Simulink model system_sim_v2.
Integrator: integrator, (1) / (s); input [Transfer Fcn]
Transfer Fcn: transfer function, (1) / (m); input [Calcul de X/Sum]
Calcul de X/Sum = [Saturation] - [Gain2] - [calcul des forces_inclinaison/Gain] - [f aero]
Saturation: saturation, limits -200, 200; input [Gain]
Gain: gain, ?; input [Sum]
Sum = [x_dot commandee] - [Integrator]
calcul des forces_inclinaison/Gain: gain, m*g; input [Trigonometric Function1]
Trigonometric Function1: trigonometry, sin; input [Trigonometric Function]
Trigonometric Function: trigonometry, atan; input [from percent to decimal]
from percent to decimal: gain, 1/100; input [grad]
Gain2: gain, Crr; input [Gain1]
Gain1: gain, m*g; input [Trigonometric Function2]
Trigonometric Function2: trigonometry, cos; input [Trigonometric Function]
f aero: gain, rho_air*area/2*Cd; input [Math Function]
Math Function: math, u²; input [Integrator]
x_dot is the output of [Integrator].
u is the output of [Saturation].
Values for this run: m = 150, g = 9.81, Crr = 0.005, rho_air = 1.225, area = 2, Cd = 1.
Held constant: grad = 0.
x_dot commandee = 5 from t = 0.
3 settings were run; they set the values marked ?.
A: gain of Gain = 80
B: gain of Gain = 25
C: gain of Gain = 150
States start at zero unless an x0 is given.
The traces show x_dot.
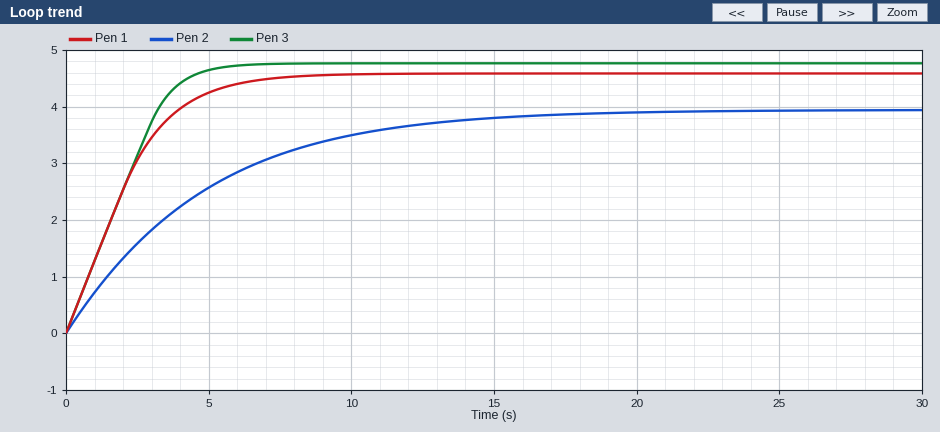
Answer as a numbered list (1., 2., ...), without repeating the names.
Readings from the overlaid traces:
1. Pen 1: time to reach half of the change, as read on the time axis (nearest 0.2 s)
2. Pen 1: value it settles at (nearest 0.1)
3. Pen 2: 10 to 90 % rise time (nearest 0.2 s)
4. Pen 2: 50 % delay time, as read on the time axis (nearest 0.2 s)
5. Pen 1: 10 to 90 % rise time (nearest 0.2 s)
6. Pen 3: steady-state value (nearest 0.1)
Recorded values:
1. 1.8 s
2. 4.6
3. 10.0 s
4. 3.4 s
5. 4.2 s
6. 4.8
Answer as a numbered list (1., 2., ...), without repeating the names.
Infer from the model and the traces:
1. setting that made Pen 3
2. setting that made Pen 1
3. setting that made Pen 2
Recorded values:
1. C
2. A
3. B
